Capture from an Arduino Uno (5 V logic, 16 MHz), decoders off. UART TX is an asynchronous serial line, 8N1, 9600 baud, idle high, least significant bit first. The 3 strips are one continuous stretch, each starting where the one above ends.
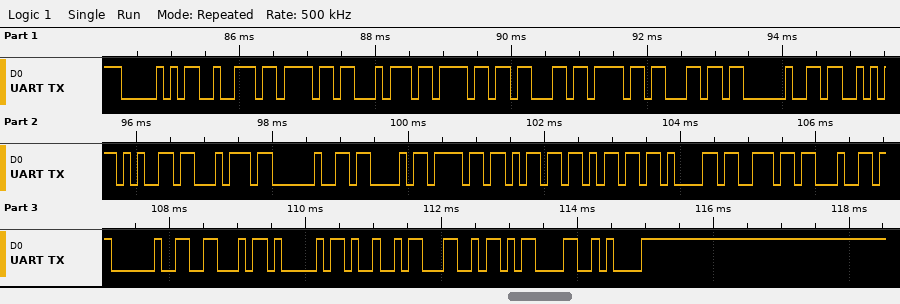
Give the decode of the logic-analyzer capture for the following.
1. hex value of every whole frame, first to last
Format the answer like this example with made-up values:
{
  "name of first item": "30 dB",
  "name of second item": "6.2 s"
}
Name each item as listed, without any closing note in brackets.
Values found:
{
  "hex value of every whole frame, first to last": "50 72 6F 74 6F 63 6F 6C 20 53 65 74 20 43 6F 6D 6D 61 6E 64 20 46 41 49 4C 0D 0A"
}
